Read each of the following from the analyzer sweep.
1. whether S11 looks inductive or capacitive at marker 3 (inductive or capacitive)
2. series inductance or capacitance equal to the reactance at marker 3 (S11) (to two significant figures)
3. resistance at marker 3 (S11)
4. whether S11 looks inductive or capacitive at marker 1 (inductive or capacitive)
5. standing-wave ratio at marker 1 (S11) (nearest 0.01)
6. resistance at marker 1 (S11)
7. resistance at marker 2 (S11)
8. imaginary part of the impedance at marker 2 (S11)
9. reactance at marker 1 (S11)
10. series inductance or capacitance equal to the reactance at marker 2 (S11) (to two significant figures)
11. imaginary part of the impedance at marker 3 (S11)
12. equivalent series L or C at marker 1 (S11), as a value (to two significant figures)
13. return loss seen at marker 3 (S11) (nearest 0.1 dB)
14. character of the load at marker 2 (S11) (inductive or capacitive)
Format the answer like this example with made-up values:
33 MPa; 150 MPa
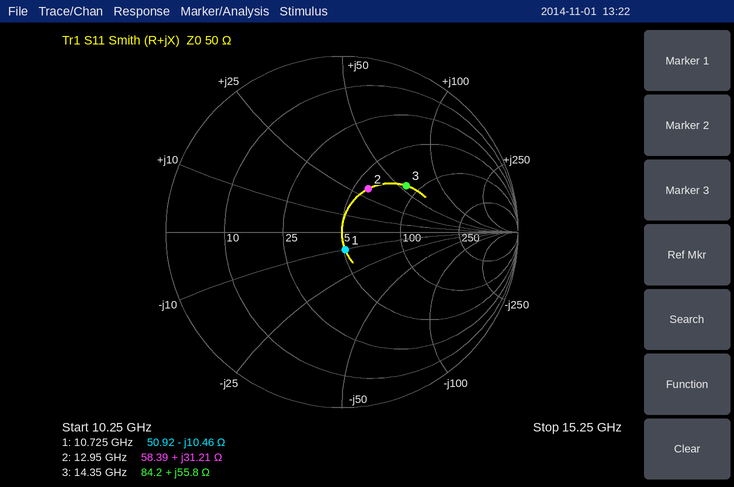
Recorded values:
inductive; 620 pH; 84.2 Ω; capacitive; 1.23; 50.92 Ω; 58.39 Ω; +31.21 Ω; -10.46 Ω; 380 pH; +55.8 Ω; 1.4 pF; 6.9 dB; inductive
